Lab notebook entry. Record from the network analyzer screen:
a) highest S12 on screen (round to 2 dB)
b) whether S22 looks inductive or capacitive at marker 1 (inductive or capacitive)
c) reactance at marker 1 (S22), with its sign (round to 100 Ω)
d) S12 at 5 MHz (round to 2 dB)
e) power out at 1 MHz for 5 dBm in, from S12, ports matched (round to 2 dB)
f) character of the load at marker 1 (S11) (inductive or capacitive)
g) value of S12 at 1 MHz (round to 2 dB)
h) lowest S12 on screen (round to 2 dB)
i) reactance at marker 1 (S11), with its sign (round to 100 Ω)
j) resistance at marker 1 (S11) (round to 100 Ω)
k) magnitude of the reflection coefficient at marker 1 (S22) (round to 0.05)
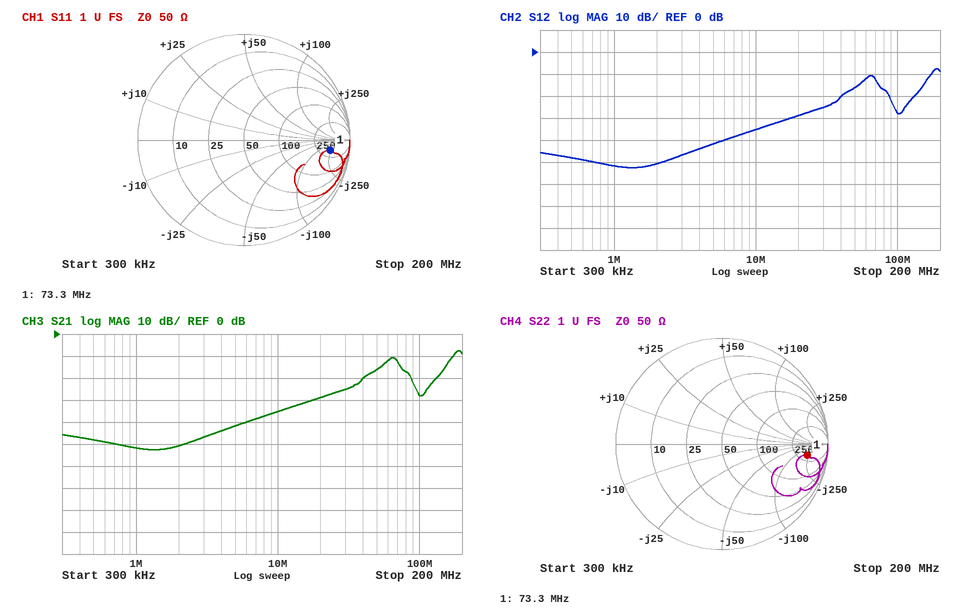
-8 dB
capacitive
-200 Ω
-42 dB
-46 dBm
capacitive
-52 dB
-52 dB
-200 Ω
400 Ω
0.80
